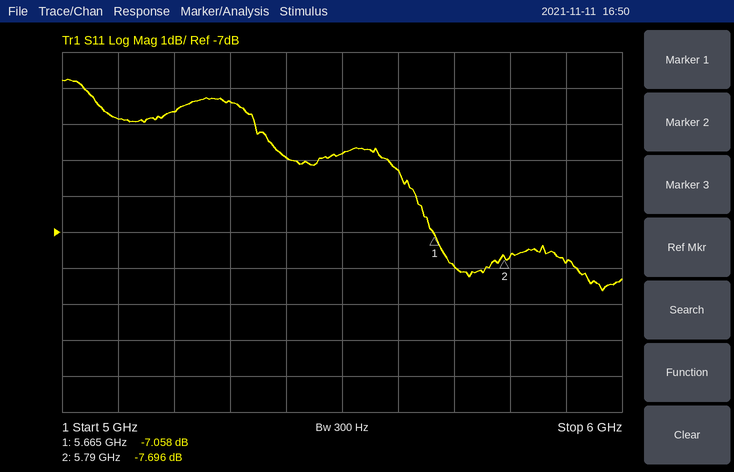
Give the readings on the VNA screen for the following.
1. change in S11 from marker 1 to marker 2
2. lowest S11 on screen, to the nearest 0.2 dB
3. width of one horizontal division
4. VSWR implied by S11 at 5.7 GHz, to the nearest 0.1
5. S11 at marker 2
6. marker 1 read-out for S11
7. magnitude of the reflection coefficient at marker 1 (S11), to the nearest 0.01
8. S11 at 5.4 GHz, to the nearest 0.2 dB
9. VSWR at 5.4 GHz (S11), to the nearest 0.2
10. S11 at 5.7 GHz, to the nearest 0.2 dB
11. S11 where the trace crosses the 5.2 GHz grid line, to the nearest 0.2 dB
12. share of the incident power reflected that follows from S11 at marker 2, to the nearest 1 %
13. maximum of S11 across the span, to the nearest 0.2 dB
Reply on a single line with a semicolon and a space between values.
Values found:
-0.638 dB; -8.6 dB; 100 MHz; 2.3; -7.696 dB; -7.058 dB; 0.44; -5.0 dB; 3.6; -8.0 dB; -3.6 dB; 17 %; -2.8 dB
